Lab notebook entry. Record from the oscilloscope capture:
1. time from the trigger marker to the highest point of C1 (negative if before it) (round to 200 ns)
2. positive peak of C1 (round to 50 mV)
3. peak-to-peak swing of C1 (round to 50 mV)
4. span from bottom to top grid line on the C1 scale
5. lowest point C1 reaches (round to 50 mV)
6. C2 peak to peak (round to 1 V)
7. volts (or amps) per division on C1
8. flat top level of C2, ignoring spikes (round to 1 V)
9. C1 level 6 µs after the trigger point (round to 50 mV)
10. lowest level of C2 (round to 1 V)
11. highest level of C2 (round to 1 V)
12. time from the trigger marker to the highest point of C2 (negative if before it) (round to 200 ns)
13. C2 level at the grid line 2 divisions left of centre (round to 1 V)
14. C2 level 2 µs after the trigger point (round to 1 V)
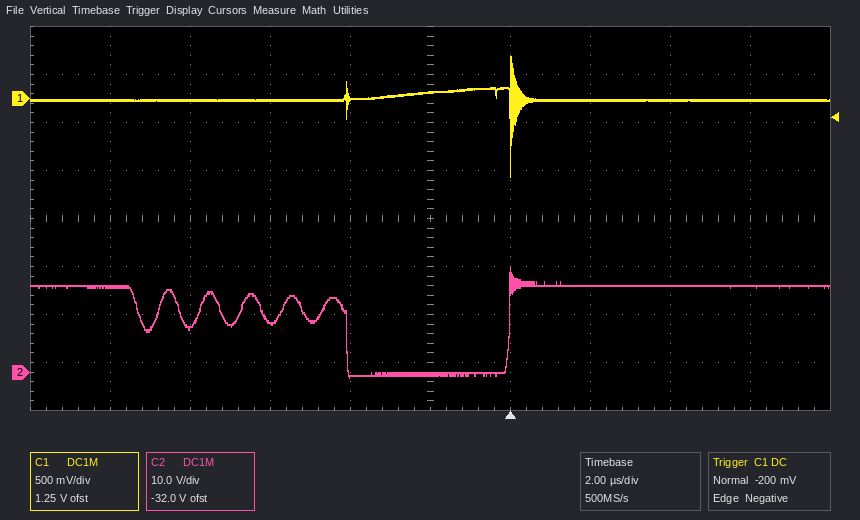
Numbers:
0.0 µs
450 mV
1.25 V
4 V
-800 mV
23 V
500 mV
18 V
0 mV
-1 V
22 V
0.0 µs
11 V
18 V
